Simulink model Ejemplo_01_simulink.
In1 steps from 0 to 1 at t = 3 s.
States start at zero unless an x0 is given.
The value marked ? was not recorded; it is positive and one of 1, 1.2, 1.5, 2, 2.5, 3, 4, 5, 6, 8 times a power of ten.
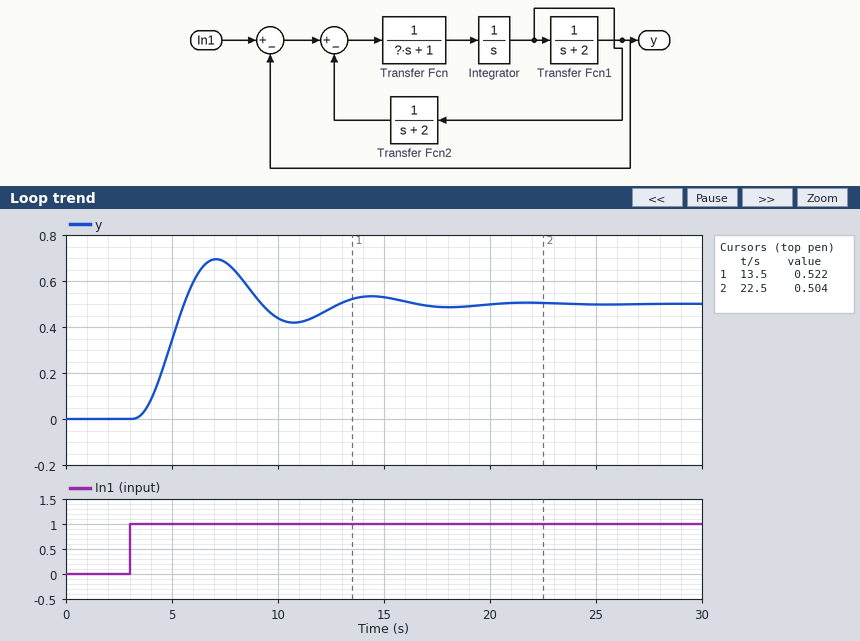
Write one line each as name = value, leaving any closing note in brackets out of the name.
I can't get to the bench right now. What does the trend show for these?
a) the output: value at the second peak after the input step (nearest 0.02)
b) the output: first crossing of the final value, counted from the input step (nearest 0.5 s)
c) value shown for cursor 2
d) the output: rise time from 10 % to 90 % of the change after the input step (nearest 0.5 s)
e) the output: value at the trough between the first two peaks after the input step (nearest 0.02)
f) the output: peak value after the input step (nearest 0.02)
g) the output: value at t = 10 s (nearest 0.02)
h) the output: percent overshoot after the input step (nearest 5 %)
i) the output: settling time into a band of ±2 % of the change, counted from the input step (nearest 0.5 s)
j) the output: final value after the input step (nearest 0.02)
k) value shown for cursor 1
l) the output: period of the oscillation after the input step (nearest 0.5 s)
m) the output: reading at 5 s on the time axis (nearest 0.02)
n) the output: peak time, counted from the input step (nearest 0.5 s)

the output: value at the second peak after the input step = 0.54
the output: first crossing of the final value, counted from the input step = 2.5 s
value shown for cursor 2 = 0.504
the output: rise time from 10 % to 90 % of the change after the input step = 1.5 s
the output: value at the trough between the first two peaks after the input step = 0.42
the output: peak value after the input step = 0.70
the output: value at t = 10 s = 0.44
the output: percent overshoot after the input step = 40 %
the output: settling time into a band of ±2 % of the change, counted from the input step = 16.0 s
the output: final value after the input step = 0.50
value shown for cursor 1 = 0.522
the output: period of the oscillation after the input step = 7.5 s
the output: reading at 5 s on the time axis = 0.34
the output: peak time, counted from the input step = 4.0 s
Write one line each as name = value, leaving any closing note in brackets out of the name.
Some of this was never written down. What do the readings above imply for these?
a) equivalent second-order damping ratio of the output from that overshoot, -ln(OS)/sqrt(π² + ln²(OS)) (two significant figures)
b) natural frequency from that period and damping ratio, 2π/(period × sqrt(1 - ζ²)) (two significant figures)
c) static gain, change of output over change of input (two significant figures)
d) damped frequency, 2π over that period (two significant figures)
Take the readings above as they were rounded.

equivalent second-order damping ratio of the output from that overshoot, -ln(OS)/sqrt(π² + ln²(OS)) = 0.28
natural frequency from that period and damping ratio, 2π/(period × sqrt(1 - ζ²)) = 0.87 rad/s
static gain, change of output over change of input = 0.50
damped frequency, 2π over that period = 0.84 rad/s
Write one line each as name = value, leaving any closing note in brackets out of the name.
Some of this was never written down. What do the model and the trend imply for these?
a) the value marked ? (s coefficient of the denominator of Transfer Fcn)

the value marked ? = 1
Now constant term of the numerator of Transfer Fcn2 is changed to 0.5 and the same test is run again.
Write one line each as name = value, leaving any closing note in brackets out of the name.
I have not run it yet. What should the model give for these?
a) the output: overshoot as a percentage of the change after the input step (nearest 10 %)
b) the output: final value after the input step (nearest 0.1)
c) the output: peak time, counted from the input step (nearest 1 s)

the output: overshoot as a percentage of the change after the input step = 30 %
the output: final value after the input step = 0.7
the output: peak time, counted from the input step = 5 s
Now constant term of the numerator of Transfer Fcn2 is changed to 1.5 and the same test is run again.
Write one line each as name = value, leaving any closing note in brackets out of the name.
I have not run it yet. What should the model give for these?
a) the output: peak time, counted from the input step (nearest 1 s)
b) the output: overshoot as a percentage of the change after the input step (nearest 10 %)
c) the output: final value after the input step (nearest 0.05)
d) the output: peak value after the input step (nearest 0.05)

the output: peak time, counted from the input step = 4 s
the output: overshoot as a percentage of the change after the input step = 50 %
the output: final value after the input step = 0.40
the output: peak value after the input step = 0.60
